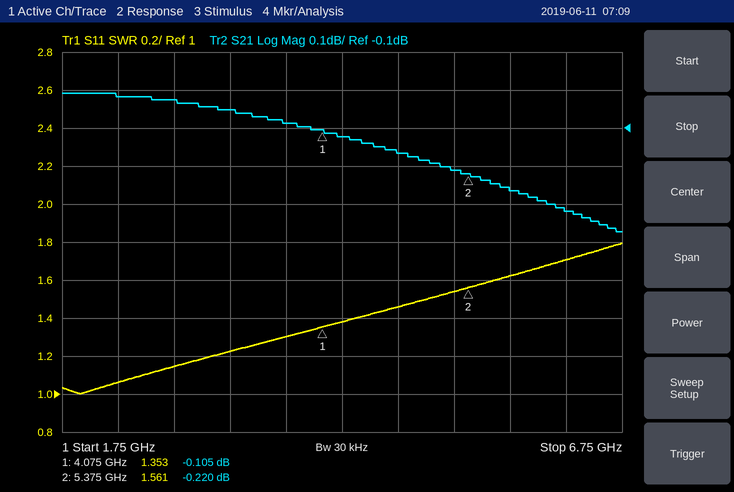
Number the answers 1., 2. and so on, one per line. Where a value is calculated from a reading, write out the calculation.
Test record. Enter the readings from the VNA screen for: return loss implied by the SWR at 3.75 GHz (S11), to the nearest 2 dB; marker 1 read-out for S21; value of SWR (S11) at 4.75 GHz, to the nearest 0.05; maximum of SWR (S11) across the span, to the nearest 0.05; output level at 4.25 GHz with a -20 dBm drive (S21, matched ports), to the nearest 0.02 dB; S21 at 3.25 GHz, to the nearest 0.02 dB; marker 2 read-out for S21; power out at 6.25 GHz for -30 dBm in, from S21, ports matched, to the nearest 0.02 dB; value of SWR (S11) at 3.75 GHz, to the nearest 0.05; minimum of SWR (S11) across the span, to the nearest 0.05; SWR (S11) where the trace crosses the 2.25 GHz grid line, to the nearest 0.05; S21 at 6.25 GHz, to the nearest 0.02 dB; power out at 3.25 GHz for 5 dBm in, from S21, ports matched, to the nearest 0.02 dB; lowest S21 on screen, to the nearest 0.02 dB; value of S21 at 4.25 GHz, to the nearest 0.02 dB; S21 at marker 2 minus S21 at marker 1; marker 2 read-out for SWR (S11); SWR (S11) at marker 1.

1. −20 log10((1.3 − 1)/(1.3 + 1)) ≈ 18 dB
2. -0.105 dB
3. 1.45
4. 1.80
5. -20 dBm + (-0.12 dB) = -20.12 dBm
6. -0.06 dB
7. -0.220 dB
8. -30 dBm + (-0.32 dB) = -30.32 dBm
9. 1.30
10. 1.00
11. 1.05
12. -0.32 dB
13. 5 dBm + (-0.06 dB) = 4.94 dBm
14. -0.38 dB
15. -0.12 dB
16. -0.22 − (-0.105) = -0.115 dB
17. 1.561
18. 1.353
